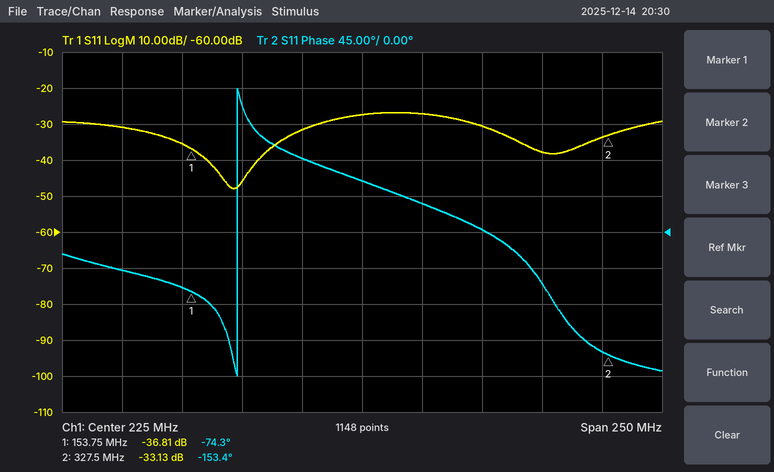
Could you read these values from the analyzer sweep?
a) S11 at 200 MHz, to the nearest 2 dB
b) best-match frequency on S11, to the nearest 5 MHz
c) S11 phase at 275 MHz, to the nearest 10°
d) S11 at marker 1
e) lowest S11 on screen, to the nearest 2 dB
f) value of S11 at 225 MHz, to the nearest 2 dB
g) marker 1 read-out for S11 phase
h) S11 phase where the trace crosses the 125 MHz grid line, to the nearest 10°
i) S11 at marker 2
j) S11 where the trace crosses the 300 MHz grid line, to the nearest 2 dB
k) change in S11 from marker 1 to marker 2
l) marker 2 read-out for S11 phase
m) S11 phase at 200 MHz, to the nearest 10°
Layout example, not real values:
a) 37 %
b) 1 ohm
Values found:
a) -32 dB
b) 170 MHz
c) 0°
d) -36.81 dB
e) -48 dB
f) -28 dB
g) -74.3°
h) -50°
i) -33.13 dB
j) -38 dB
k) 3.68 dB
l) -153.4°
m) 90°
